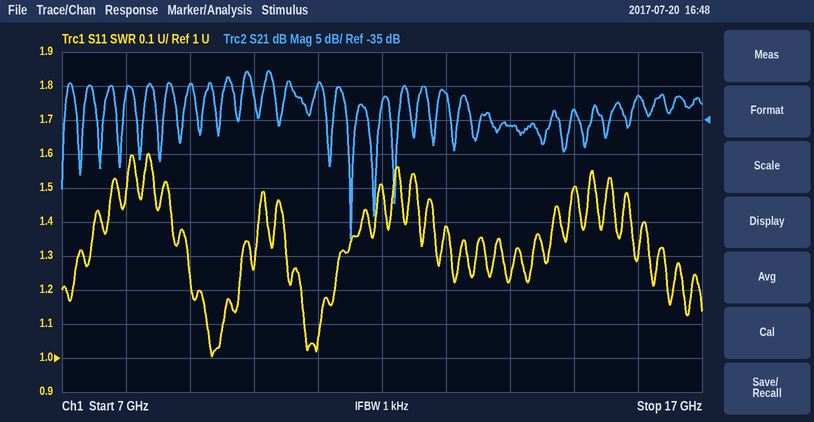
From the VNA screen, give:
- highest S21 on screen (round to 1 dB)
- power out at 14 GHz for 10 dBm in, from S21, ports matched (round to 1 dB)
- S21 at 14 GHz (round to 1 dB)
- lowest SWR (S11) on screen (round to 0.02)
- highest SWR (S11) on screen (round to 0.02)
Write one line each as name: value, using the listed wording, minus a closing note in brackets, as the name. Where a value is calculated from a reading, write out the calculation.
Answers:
highest S21 on screen: -28 dB
power out at 14 GHz for 10 dBm in, from S21, ports matched: 10 dBm + (-36 dB) = -26 dBm
S21 at 14 GHz: -36 dB
lowest SWR (S11) on screen: 1.00
highest SWR (S11) on screen: 1.60
